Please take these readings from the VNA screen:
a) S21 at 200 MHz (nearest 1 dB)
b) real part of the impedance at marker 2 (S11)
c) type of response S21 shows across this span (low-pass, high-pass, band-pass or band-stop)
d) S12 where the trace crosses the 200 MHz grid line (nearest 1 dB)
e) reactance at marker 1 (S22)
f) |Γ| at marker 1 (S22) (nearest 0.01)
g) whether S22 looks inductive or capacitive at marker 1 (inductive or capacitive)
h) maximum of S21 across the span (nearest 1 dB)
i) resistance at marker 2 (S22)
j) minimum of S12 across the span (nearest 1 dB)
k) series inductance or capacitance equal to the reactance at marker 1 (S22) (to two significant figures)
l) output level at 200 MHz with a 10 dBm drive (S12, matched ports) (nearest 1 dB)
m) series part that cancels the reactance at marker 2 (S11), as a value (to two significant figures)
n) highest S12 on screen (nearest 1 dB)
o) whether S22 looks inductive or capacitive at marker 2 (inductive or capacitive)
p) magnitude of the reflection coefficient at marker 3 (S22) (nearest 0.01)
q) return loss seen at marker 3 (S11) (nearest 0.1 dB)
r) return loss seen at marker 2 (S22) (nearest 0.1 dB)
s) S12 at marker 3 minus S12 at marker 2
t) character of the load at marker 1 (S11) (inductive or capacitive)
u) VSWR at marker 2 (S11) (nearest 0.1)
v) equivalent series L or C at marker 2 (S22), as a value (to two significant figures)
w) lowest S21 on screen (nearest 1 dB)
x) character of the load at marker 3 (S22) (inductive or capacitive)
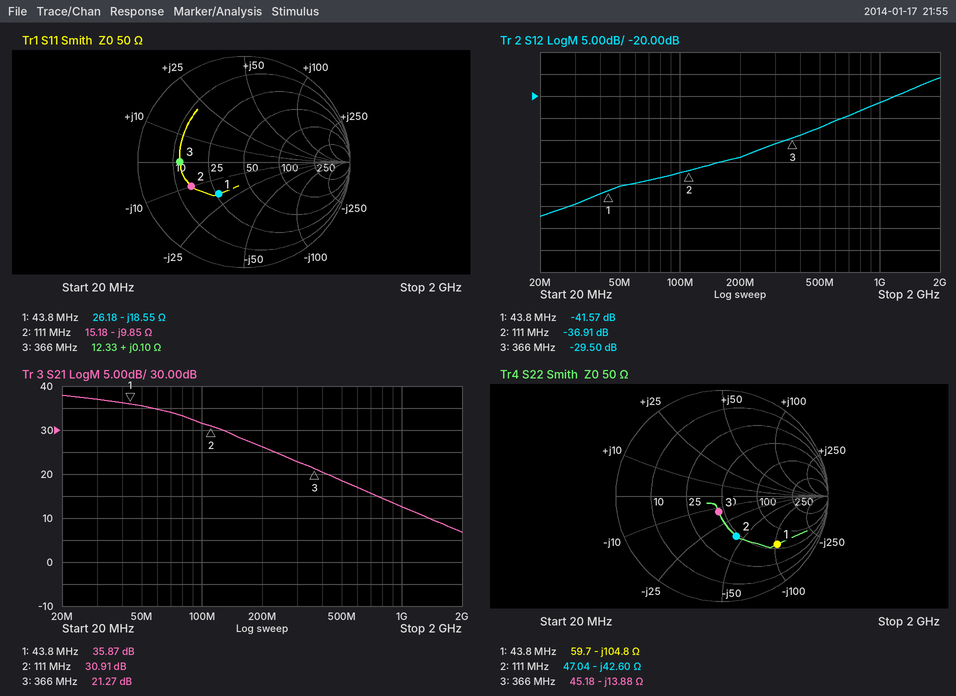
26 dB
15.18 Ω
low-pass
-34 dB
-104.8 Ω
0.69
capacitive
38 dB
47.04 Ω
-47 dB
35 pF
-24 dBm
14 nH
-16 dB
capacitive
0.15
4.4 dB
7.9 dB
7.41 dB
capacitive
3.4
34 pF
7 dB
capacitive
